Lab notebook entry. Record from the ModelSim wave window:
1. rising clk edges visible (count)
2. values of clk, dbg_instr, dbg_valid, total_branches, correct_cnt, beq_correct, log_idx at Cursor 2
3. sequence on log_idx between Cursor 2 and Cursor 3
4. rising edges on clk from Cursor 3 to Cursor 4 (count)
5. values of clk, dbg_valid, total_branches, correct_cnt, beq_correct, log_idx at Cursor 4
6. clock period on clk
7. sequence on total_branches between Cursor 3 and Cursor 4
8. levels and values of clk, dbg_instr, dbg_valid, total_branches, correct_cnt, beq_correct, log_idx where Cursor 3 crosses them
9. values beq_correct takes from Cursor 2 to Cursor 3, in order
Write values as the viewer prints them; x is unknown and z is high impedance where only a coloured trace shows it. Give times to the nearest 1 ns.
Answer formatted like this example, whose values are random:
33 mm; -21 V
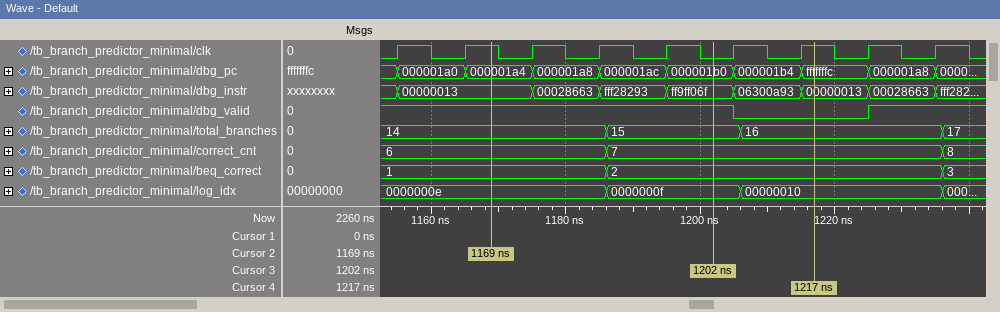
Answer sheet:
9; clk=1, dbg_instr=00000013, dbg_valid=1, total_branches=14, correct_cnt=6, beq_correct=1, log_idx=0000000e; 0000000e, 0000000f; 2; clk=1, dbg_valid=0, total_branches=16, correct_cnt=7, beq_correct=2, log_idx=00000010; 10 ns; 15, 16; clk=0, dbg_instr=ff9ff06f, dbg_valid=1, total_branches=15, correct_cnt=7, beq_correct=2, log_idx=0000000f; 1, 2
